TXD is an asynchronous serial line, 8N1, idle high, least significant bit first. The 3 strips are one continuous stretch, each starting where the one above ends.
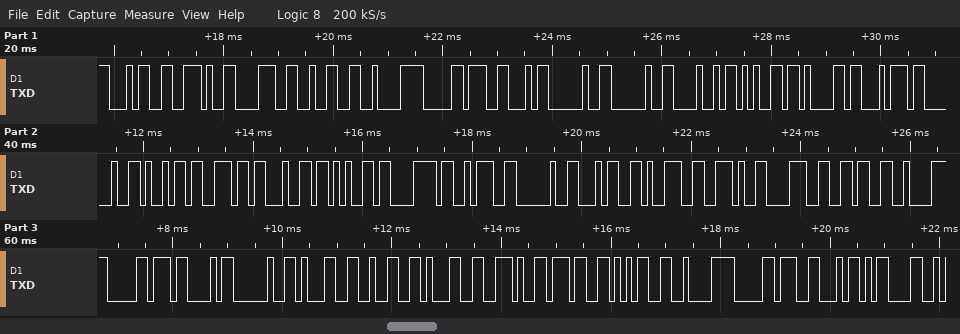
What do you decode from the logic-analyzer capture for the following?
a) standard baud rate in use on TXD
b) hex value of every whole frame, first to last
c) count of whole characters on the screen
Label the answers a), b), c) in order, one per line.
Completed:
a) 9600 baud
b) 34 2E 38 32 C2 B0 46 20 20 48 65 61 74 20 69 6E 64 65 78 3A 20 34 39 2E 38 36 C2 B0 43 20 31 32 31 2E 37 35 C2 B0 46 0D
c) 40
